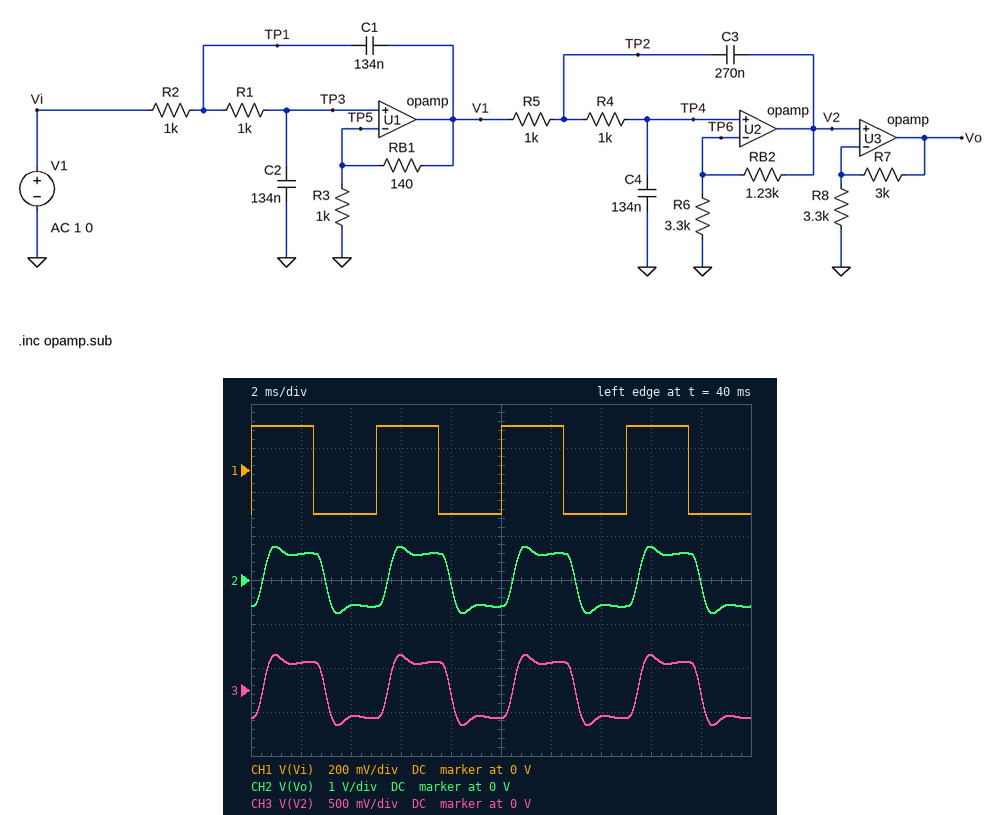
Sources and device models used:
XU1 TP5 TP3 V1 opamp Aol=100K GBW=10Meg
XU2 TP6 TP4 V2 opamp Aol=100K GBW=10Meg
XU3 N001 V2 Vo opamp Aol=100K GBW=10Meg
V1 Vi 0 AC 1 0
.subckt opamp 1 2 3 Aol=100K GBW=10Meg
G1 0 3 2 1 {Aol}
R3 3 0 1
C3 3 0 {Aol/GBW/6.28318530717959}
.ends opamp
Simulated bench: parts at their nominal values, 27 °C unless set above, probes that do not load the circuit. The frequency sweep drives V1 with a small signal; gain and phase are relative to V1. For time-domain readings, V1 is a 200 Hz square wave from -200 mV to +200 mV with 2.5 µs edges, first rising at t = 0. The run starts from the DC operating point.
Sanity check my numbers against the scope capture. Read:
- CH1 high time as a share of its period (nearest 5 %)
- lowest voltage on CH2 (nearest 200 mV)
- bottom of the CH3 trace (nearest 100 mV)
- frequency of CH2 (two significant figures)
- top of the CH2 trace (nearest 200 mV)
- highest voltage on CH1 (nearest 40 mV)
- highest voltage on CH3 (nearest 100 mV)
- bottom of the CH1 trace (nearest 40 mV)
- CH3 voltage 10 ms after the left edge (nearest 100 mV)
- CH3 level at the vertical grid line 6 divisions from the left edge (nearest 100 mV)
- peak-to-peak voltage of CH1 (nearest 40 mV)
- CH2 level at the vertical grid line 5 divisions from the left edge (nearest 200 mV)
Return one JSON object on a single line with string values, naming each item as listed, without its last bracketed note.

{"CH1 high time as a share of its period": "50 %", "lowest voltage on CH2": "-800 mV", "bottom of the CH3 trace": "-400 mV", "frequency of CH2": "200 Hz", "top of the CH2 trace": "800 mV", "highest voltage on CH1": "200 mV", "highest voltage on CH3": "400 mV", "bottom of the CH1 trace": "-200 mV", "CH3 voltage 10 ms after the left edge": "-300 mV", "CH3 level at the vertical grid line 6 divisions from the left edge": "300 mV", "peak-to-peak voltage of CH1": "400 mV", "CH2 level at the vertical grid line 5 divisions from the left edge": "-600 mV"}
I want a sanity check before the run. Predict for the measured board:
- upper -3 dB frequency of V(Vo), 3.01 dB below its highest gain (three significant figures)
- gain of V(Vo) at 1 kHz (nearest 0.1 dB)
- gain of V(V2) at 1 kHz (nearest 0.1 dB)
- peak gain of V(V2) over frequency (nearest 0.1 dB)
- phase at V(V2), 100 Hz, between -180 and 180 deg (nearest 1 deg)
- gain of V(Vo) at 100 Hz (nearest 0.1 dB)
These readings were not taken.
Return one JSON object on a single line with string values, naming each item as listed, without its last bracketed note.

{"upper -3 dB frequency of V(Vo), 3.01 dB below its highest gain": "874 Hz", "gain of V(Vo) at 1 kHz": "4.4 dB", "gain of V(V2) at 1 kHz": "-1.3 dB", "peak gain of V(V2) over frequency": "4.4 dB", "phase at V(V2), 100 Hz, between -180 and 180 deg": "-15 deg", "gain of V(Vo) at 100 Hz": "9.5 dB"}
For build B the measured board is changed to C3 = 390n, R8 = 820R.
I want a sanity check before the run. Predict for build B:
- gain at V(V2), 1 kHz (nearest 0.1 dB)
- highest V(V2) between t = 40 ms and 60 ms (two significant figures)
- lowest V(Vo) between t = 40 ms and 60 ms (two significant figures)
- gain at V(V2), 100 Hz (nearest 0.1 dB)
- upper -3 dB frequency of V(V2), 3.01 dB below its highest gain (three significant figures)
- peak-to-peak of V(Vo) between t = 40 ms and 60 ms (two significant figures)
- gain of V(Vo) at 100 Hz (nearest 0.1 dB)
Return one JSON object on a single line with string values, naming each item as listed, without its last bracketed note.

{"gain at V(V2), 1 kHz": "-2.5 dB", "highest V(V2) between t = 40 ms and 60 ms": "520 mV", "lowest V(Vo) between t = 40 ms and 60 ms": "-2.4 V", "gain at V(V2), 100 Hz": "4.0 dB", "upper -3 dB frequency of V(V2), 3.01 dB below its highest gain": "784 Hz", "peak-to-peak of V(Vo) between t = 40 ms and 60 ms": "4.8 V", "gain of V(Vo) at 100 Hz": "17.4 dB"}
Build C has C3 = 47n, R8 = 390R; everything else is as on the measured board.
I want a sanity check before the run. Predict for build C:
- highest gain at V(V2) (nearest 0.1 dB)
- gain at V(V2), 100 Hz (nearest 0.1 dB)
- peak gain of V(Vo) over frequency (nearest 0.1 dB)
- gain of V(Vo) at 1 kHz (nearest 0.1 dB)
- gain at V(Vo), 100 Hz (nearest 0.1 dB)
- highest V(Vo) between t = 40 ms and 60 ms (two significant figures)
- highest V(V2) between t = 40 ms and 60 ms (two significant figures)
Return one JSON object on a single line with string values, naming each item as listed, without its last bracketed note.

{"highest gain at V(V2)": "3.9 dB", "gain at V(V2), 100 Hz": "3.8 dB", "peak gain of V(Vo) over frequency": "22.7 dB", "gain of V(Vo) at 1 kHz": "13.8 dB", "gain at V(Vo), 100 Hz": "22.5 dB", "highest V(Vo) between t = 40 ms and 60 ms": "2.7 V", "highest V(V2) between t = 40 ms and 60 ms": "310 mV"}
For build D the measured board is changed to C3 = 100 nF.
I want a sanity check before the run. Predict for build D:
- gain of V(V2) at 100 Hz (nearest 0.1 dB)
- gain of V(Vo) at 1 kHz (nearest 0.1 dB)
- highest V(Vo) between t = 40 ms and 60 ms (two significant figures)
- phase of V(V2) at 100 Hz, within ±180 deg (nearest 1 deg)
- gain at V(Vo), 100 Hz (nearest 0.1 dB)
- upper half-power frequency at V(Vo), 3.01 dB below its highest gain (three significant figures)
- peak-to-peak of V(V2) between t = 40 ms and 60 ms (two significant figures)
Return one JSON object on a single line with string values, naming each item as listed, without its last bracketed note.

{"gain of V(V2) at 100 Hz": "3.8 dB", "gain of V(Vo) at 1 kHz": "1.8 dB", "highest V(Vo) between t = 40 ms and 60 ms": "600 mV", "phase of V(V2) at 100 Hz, within ±180 deg": "-17 deg", "gain at V(Vo), 100 Hz": "9.4 dB", "upper half-power frequency at V(Vo), 3.01 dB below its highest gain": "593 Hz", "peak-to-peak of V(V2) between t = 40 ms and 60 ms": "630 mV"}
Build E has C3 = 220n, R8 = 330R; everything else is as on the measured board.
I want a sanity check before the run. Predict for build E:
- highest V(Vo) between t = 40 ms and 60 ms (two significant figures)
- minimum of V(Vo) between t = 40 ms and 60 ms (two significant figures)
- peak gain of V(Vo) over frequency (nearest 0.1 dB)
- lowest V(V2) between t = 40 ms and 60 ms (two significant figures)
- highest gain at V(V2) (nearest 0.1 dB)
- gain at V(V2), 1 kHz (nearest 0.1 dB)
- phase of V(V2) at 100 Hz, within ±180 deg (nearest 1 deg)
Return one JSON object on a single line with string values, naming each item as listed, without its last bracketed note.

{"highest V(Vo) between t = 40 ms and 60 ms": "3.6 V", "minimum of V(Vo) between t = 40 ms and 60 ms": "-3.6 V", "peak gain of V(Vo) over frequency": "24.0 dB", "lowest V(V2) between t = 40 ms and 60 ms": "-360 mV", "highest gain at V(V2)": "3.9 dB", "gain at V(V2), 1 kHz": "-1.6 dB", "phase of V(V2) at 100 Hz, within ±180 deg": "-16 deg"}
